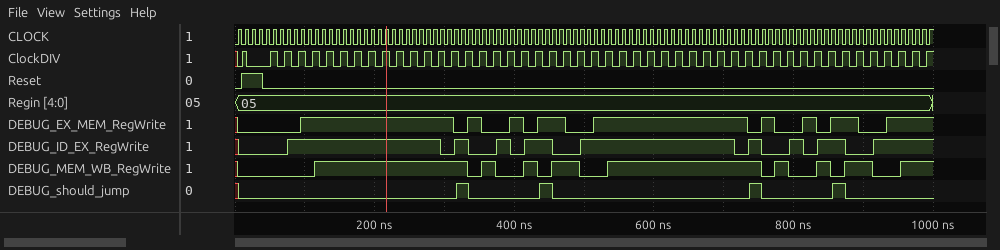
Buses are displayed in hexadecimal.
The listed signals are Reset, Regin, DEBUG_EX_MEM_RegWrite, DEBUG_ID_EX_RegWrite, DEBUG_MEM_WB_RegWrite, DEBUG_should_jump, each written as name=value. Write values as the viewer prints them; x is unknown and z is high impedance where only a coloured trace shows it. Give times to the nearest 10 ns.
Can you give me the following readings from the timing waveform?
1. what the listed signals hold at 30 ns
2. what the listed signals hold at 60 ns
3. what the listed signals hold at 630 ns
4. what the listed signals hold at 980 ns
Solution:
Reset=1, Regin=05, DEBUG_EX_MEM_RegWrite=0, DEBUG_ID_EX_RegWrite=0, DEBUG_MEM_WB_RegWrite=0, DEBUG_should_jump=0
Reset=0, Regin=05, DEBUG_EX_MEM_RegWrite=0, DEBUG_ID_EX_RegWrite=0, DEBUG_MEM_WB_RegWrite=0, DEBUG_should_jump=0
Reset=0, Regin=05, DEBUG_EX_MEM_RegWrite=1, DEBUG_ID_EX_RegWrite=1, DEBUG_MEM_WB_RegWrite=1, DEBUG_should_jump=0
Reset=0, Regin=05, DEBUG_EX_MEM_RegWrite=1, DEBUG_ID_EX_RegWrite=1, DEBUG_MEM_WB_RegWrite=1, DEBUG_should_jump=0
